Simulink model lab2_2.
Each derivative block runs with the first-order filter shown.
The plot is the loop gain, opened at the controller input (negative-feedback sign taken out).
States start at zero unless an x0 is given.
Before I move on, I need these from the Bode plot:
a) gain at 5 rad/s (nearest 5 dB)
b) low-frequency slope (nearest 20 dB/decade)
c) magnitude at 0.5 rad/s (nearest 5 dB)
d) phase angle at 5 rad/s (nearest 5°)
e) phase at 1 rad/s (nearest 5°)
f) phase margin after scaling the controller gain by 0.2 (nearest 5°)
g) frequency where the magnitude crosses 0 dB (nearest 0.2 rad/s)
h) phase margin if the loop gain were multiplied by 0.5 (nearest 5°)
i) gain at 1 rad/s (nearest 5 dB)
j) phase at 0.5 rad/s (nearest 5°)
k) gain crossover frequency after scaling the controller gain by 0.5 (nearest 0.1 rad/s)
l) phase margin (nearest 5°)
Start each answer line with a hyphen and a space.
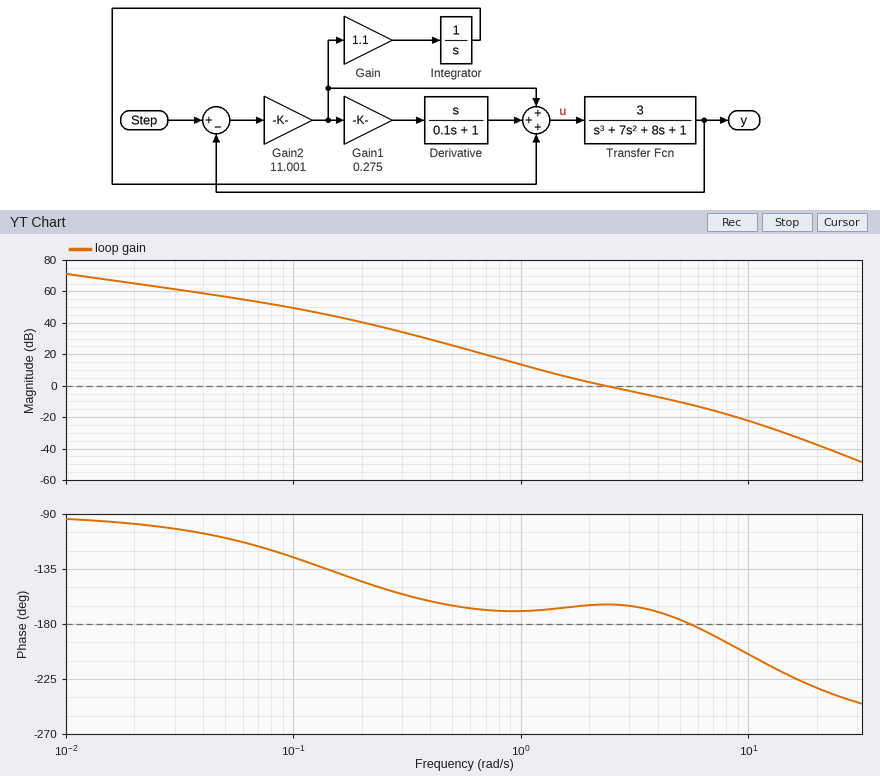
- -10 dB
- -20 dB/decade
- 25 dB
- -175°
- -170°
- 10°
- 2.4 rad/s
- 15°
- 15 dB
- -165°
- 1.6 rad/s
- 15°
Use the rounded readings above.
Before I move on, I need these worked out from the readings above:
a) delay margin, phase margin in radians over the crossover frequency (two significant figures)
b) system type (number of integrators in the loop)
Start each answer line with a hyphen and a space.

- 0.11 s
- 1
